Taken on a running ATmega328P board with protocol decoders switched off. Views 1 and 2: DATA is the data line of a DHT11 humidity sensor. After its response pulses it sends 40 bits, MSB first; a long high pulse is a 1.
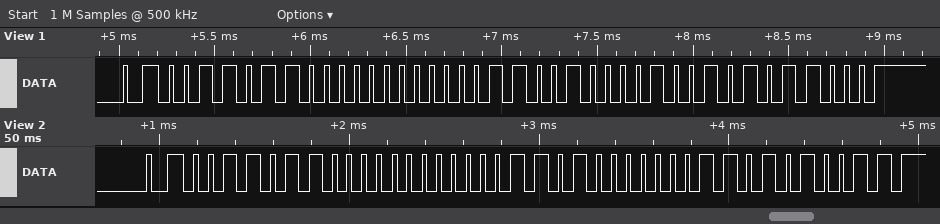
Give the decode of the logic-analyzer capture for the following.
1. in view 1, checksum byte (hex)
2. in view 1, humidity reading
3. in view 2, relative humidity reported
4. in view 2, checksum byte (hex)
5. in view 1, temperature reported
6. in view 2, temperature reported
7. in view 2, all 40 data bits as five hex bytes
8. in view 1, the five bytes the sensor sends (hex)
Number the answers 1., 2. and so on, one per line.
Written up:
1. 0x58
2. 54 %
3. 54 %
4. 0x53
5. 25.9 °C
6. 26.3 °C
7. 36 00 1A 03 53
8. 36 00 19 09 58
